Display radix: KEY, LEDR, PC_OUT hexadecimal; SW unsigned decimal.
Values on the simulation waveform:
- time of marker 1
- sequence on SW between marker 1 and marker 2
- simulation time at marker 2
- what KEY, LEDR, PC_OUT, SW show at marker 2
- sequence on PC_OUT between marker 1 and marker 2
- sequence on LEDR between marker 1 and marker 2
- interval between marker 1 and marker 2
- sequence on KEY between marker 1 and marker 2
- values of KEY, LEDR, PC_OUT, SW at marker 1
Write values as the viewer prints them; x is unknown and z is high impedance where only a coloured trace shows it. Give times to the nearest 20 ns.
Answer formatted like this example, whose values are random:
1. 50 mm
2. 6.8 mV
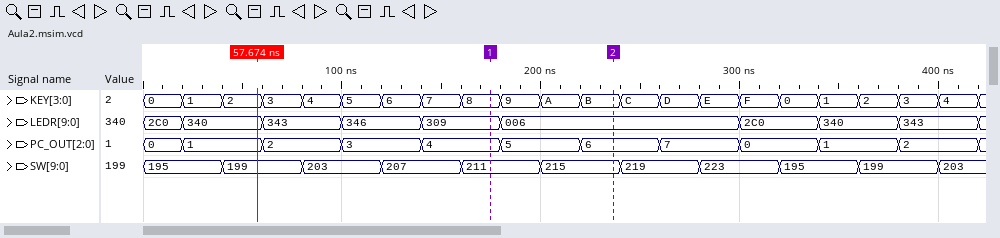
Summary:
1. 180 ns
2. 211, 215
3. 240 ns
4. KEY=B, LEDR=006, PC_OUT=6, SW=215
5. 4, 5, 6
6. 309, 006
7. 60 ns
8. 8, 9, A, B
9. KEY=8, LEDR=309, PC_OUT=4, SW=211
